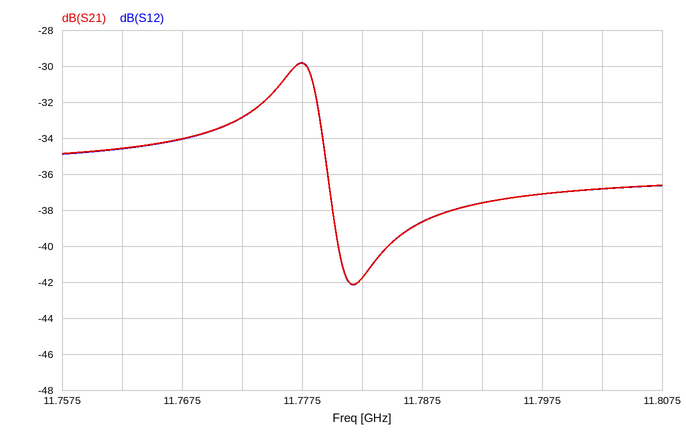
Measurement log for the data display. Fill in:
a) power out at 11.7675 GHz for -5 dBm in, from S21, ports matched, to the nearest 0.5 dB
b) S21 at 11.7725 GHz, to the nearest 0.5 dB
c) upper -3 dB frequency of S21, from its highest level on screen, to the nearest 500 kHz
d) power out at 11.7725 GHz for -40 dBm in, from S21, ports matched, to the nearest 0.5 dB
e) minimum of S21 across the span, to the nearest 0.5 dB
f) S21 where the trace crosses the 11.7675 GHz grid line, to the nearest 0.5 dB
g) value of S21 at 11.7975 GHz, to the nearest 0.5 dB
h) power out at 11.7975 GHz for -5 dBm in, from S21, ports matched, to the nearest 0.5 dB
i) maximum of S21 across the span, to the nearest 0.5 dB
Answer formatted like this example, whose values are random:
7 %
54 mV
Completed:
-39.0 dBm
-33.0 dB
11.7790 GHz
-73.0 dBm
-42.0 dB
-34.0 dB
-37.0 dB
-42.0 dBm
-30.0 dB
